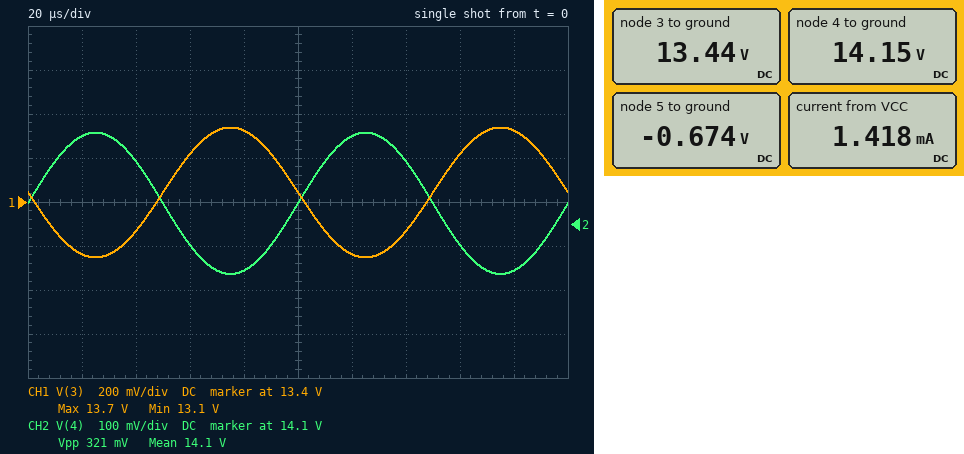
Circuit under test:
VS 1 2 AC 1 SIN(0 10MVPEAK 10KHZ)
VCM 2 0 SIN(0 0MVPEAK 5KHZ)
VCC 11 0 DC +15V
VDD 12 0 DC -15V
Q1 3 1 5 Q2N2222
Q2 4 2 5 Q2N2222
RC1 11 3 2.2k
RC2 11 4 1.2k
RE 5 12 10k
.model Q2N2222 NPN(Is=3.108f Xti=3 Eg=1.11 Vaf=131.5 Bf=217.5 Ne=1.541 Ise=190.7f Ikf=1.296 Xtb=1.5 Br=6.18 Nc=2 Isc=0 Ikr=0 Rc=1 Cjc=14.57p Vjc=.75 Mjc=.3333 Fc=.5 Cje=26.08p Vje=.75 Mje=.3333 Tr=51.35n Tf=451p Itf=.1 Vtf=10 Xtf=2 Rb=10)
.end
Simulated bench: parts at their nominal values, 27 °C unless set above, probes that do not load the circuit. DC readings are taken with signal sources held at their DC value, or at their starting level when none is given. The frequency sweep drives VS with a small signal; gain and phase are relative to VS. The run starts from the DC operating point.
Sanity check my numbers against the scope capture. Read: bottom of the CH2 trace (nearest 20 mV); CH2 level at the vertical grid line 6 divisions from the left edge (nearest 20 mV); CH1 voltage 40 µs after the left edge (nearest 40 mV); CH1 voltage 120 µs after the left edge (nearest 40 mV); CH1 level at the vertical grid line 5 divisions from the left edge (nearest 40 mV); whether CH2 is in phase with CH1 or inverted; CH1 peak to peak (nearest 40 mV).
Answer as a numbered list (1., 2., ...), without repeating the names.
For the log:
1. 13.98 V
2. 14.30 V
3. 13.28 V
4. 13.16 V
5. 13.44 V
6. inverted
7. 600 mV
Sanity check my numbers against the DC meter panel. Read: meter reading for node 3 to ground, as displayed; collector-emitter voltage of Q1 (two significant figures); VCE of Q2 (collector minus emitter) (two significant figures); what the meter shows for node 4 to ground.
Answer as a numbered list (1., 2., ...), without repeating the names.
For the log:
1. 13.44 V
2. 14 V
3. 15 V
4. 14.15 V
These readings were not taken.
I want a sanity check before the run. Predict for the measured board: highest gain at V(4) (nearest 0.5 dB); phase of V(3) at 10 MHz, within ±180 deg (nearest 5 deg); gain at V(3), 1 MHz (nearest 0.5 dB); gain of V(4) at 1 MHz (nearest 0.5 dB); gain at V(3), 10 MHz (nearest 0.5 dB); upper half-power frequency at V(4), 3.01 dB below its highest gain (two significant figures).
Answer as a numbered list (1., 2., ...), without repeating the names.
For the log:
1. 24.0 dB
2. 135 deg
3. 29.5 dB
4. 24.0 dB
5. 27.0 dB
6. 18 MHz
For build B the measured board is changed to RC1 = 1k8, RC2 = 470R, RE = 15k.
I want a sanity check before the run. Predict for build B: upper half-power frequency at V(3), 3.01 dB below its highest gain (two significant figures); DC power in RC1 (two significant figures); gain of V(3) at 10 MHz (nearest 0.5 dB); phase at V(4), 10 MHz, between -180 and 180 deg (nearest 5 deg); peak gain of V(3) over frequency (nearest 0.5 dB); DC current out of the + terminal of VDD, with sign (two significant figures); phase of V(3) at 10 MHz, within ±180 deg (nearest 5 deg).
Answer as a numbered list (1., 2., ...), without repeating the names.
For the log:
1. 15 MHz
2. 400 µW
3. 22.5 dB
4. -15 deg
5. 24.5 dB
6. -960 µA
7. 140 deg
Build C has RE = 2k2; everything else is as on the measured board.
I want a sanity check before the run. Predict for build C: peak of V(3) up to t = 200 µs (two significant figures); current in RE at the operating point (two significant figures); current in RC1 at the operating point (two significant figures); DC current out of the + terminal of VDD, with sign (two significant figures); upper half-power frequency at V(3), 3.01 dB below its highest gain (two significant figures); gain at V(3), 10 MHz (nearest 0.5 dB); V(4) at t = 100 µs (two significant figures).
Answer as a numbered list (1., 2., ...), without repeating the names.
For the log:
1. 9.3 V
2. 6.5 mA
3. 3.2 mA
4. -6.5 mA
5. 6.1 MHz
6. 36.5 dB
7. 11 V
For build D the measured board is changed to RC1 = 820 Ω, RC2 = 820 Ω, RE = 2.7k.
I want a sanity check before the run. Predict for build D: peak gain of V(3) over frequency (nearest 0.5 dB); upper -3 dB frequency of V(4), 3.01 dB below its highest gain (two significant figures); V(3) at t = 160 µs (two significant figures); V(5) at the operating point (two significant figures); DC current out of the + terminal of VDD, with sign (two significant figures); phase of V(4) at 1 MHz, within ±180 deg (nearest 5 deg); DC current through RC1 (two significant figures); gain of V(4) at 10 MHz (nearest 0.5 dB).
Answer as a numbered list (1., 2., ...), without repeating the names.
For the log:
1. 32.0 dB
2. 17 MHz
3. 13 V
4. -710 mV
5. -5.3 mA
6. -5 deg
7. 2.6 mA
8. 31.0 dB
